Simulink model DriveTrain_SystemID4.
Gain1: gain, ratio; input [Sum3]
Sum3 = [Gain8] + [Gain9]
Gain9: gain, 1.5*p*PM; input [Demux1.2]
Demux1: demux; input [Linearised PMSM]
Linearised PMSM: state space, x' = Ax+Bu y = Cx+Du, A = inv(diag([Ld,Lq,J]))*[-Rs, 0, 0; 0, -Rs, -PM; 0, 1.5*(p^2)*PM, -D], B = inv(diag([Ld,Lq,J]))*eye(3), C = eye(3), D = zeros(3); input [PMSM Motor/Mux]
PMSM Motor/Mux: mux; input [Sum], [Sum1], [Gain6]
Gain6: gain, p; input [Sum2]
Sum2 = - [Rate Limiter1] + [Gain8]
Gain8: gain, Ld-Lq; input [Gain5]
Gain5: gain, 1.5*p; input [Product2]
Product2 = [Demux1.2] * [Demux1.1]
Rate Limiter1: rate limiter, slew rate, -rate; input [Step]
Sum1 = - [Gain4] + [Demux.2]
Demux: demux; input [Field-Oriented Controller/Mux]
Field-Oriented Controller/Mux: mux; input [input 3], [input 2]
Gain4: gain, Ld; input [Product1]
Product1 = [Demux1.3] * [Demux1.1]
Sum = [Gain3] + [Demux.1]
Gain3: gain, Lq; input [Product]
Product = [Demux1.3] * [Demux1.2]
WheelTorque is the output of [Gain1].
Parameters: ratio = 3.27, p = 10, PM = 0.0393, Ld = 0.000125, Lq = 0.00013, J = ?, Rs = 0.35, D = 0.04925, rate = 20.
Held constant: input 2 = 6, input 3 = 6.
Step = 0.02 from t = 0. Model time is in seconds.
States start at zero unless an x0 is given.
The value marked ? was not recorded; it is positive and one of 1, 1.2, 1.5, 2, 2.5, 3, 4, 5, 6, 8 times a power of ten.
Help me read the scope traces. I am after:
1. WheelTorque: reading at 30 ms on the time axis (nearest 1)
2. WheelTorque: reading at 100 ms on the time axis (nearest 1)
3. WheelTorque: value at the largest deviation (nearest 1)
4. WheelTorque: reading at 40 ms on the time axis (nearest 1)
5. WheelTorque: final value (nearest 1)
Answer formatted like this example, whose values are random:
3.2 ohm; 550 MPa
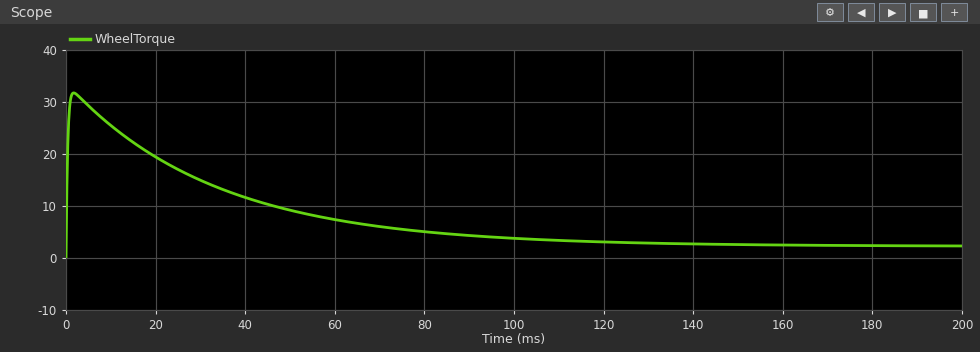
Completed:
15; 4; 32; 12; 2
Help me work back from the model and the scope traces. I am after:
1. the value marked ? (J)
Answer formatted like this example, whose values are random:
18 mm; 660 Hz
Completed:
0.025
